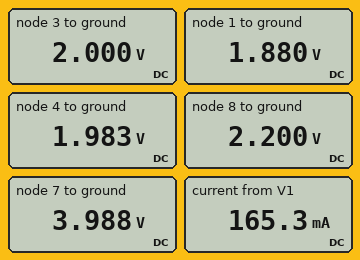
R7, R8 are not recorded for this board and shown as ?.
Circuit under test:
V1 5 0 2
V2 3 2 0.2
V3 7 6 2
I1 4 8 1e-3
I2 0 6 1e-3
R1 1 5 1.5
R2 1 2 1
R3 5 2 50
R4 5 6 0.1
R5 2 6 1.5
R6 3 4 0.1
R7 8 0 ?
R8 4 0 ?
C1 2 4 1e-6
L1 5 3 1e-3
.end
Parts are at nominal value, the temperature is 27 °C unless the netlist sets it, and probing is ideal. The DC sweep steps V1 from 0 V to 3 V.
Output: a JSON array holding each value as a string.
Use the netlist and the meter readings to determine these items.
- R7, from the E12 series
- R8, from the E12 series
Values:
["2.2 kΩ", "12 Ω"]
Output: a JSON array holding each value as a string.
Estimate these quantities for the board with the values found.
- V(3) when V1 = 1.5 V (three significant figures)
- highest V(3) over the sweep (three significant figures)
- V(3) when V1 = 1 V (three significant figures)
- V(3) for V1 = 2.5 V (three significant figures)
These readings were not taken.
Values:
["1.50 V", "3.00 V", "1.00 V", "2.50 V"]
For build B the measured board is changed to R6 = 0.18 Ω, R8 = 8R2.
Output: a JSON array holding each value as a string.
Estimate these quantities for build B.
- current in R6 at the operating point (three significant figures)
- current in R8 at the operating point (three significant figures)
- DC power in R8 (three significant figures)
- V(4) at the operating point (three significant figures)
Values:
["240 mA", "239 mA", "467 mW", "1.96 V"]
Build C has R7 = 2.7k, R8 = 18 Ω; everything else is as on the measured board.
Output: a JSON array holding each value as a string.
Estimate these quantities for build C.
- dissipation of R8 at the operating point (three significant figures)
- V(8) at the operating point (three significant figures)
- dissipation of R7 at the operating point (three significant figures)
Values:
["220 mW", "2.70 V", "2.70 mW"]
